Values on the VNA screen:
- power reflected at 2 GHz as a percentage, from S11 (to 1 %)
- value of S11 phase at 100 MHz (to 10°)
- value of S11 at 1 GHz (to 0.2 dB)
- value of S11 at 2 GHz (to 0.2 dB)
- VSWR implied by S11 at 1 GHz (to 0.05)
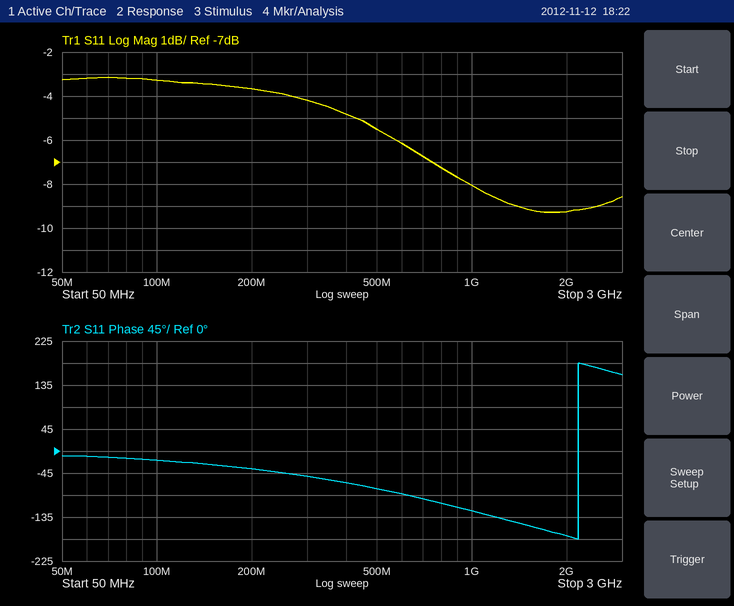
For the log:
12 %
-20°
-8.0 dB
-9.2 dB
2.30
